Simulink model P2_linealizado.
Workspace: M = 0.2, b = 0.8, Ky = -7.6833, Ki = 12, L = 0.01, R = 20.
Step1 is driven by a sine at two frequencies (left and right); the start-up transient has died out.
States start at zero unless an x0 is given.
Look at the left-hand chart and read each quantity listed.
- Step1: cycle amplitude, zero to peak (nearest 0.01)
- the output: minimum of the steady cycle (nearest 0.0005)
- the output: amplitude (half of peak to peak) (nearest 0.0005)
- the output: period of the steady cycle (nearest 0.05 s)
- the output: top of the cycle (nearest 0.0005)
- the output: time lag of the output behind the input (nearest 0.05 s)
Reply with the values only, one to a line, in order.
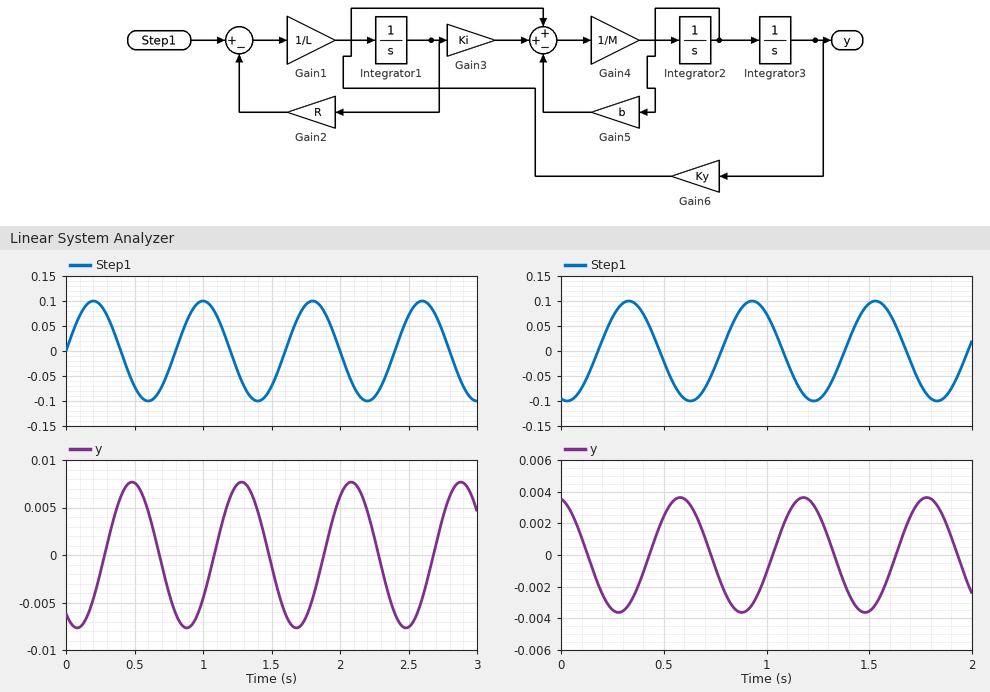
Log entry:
0.10
-0.0075
0.0075
0.80 s
0.0075
0.30 s
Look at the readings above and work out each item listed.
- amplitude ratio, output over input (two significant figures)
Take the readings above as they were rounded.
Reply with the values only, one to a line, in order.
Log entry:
0.075
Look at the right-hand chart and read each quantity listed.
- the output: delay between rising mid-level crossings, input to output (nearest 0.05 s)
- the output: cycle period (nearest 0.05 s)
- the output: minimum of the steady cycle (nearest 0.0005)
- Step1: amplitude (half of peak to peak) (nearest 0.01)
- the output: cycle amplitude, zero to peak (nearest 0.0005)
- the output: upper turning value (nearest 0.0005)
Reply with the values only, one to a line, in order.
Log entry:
0.25 s
0.60 s
-0.0035
0.10
0.0035
0.0035
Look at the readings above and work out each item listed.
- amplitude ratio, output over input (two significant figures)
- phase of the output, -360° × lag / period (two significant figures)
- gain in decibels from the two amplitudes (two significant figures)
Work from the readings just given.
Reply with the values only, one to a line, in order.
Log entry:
0.035
-150°
-29 dB
